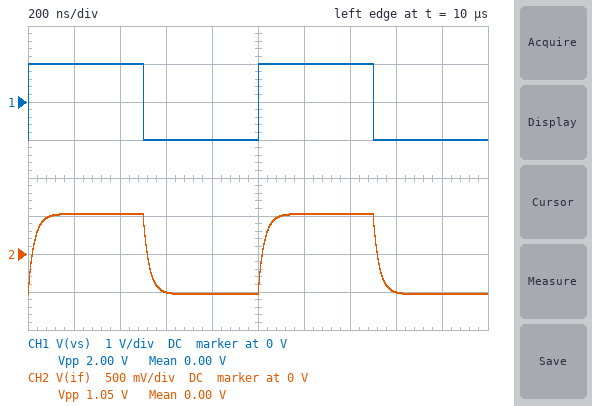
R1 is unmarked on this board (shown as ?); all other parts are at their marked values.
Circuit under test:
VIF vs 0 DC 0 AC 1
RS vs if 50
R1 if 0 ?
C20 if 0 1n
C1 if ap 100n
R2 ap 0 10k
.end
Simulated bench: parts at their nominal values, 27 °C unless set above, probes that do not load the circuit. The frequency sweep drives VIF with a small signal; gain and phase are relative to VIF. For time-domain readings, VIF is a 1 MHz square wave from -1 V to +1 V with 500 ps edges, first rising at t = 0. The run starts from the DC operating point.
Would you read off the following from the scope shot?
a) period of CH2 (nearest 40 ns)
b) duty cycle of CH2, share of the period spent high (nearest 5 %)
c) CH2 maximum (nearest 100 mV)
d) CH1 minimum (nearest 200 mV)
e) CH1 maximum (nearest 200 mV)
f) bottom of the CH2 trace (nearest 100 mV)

1.00 µs
50 %
500 mV
-1.0 V
1.0 V
-500 mV
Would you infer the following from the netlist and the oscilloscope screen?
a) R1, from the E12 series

56 Ω
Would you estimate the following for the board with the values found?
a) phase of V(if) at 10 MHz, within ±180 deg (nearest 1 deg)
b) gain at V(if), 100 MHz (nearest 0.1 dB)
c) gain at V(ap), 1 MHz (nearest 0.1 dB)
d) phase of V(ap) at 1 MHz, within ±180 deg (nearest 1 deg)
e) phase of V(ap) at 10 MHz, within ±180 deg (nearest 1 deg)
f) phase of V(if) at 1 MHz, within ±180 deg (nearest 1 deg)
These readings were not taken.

-59 deg
-30.0 dB
-5.7 dB
-9 deg
-59 deg
-9 deg
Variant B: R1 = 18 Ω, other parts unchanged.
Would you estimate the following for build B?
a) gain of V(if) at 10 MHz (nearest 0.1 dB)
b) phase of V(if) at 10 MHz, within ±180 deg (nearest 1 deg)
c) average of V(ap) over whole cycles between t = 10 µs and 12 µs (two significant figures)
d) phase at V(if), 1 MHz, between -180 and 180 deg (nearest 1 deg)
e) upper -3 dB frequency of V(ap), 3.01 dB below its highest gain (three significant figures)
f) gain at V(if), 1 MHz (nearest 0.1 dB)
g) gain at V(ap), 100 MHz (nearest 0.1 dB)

-13.8 dB
-40 deg
260 mV
-5 deg
12.0 MHz
-11.6 dB
-30.0 dB
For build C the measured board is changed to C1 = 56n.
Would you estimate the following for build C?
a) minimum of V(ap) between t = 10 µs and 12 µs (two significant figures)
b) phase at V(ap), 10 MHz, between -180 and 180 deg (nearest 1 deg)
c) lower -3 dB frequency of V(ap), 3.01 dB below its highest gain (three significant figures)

-11 mV
-59 deg
283 Hz
